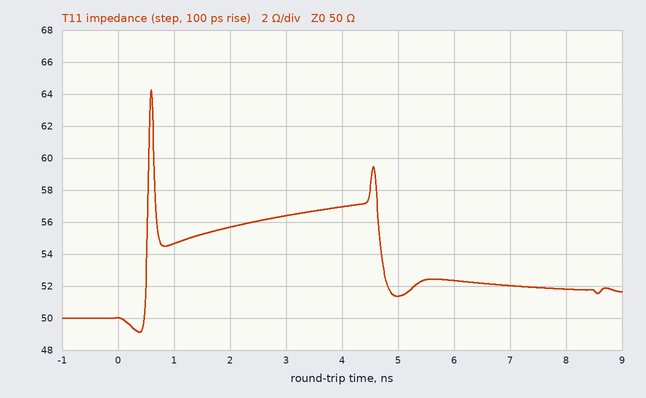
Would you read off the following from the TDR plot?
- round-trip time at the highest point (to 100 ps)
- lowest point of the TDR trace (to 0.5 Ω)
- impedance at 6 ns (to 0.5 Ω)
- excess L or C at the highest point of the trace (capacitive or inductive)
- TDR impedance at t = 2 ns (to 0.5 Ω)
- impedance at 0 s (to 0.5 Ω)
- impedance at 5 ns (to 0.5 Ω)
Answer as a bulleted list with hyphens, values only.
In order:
- 600 ps
- 49.0 Ω
- 52.5 Ω
- inductive
- 55.5 Ω
- 50.0 Ω
- 51.5 Ω
